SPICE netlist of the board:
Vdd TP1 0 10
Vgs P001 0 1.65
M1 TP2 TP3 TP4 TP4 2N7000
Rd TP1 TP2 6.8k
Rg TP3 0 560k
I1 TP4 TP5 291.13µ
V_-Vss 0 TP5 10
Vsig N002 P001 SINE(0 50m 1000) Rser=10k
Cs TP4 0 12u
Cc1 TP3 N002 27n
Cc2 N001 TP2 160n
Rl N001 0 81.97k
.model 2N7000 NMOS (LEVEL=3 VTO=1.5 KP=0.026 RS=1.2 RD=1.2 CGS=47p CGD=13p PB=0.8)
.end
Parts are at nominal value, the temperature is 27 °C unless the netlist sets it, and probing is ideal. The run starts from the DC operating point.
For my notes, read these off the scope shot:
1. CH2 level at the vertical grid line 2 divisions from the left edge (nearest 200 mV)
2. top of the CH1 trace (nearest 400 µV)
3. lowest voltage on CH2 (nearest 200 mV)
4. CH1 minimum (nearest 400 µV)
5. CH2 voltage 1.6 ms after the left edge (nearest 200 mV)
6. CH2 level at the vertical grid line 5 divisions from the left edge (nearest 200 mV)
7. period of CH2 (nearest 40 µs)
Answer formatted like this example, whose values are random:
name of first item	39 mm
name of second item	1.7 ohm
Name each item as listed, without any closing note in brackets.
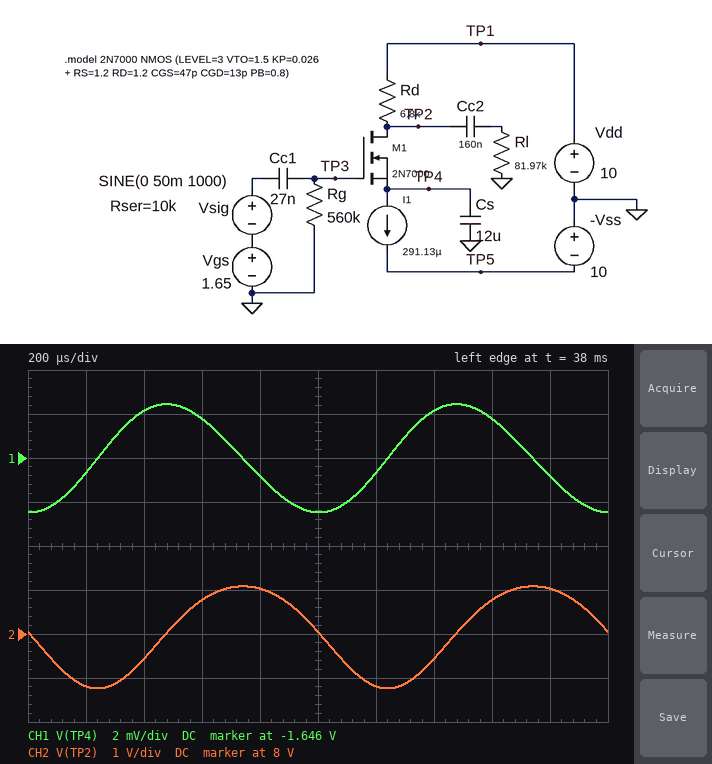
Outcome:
CH2 level at the vertical grid line 2 divisions from the left edge	7.4 V
top of the CH1 trace	-1.6436 V
lowest voltage on CH2	6.8 V
CH1 minimum	-1.6484 V
CH2 voltage 1.6 ms after the left edge	8.8 V
CH2 level at the vertical grid line 5 divisions from the left edge	8.0 V
period of CH2	1.00 ms
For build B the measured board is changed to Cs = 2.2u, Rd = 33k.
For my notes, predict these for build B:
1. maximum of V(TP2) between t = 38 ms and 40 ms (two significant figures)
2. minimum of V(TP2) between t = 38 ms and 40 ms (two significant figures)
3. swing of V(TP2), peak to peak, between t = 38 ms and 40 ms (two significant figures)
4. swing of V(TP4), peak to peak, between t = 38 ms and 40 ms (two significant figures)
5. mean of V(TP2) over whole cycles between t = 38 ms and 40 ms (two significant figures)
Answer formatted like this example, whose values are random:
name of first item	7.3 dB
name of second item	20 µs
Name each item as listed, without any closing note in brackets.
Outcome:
maximum of V(TP2) between t = 38 ms and 40 ms	3.6 V
minimum of V(TP2) between t = 38 ms and 40 ms	-1.6 V
swing of V(TP2), peak to peak, between t = 38 ms and 40 ms	5.1 V
swing of V(TP4), peak to peak, between t = 38 ms and 40 ms	18 mV
mean of V(TP2) over whole cycles between t = 38 ms and 40 ms	390 mV
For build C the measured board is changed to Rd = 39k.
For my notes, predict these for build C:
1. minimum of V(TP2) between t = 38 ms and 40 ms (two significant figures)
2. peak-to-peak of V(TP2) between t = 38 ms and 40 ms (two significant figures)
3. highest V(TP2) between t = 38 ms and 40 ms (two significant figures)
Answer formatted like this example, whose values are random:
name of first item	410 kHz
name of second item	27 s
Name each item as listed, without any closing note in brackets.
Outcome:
minimum of V(TP2) between t = 38 ms and 40 ms	-1.6 V
peak-to-peak of V(TP2) between t = 38 ms and 40 ms	1.9 V
highest V(TP2) between t = 38 ms and 40 ms	240 mV
